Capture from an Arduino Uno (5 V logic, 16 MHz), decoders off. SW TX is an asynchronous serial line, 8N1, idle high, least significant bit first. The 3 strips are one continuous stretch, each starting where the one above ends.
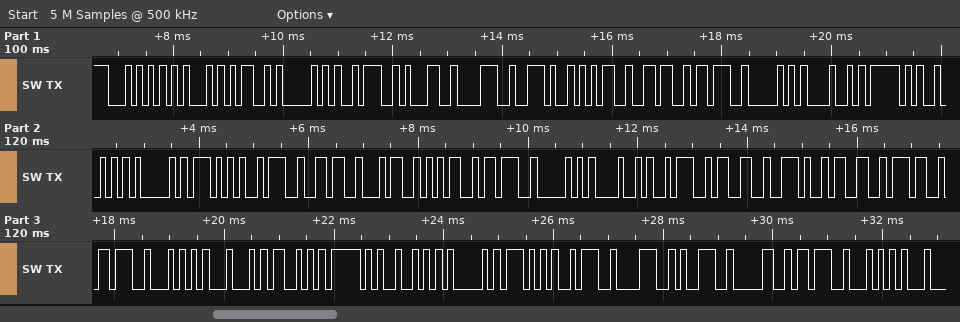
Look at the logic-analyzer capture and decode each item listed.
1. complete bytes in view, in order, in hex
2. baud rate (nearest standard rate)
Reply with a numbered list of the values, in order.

1. 54 45 4D 50 3A 31 38 2E 35 36 3B 50 48 5F 52 41 57 3A 36 34 35 3B 50 48 3A 33 2E 33 37 3B 54 44 53 5F 52 41 57 3A 38 39 30 3B 54
2. 9600 baud
